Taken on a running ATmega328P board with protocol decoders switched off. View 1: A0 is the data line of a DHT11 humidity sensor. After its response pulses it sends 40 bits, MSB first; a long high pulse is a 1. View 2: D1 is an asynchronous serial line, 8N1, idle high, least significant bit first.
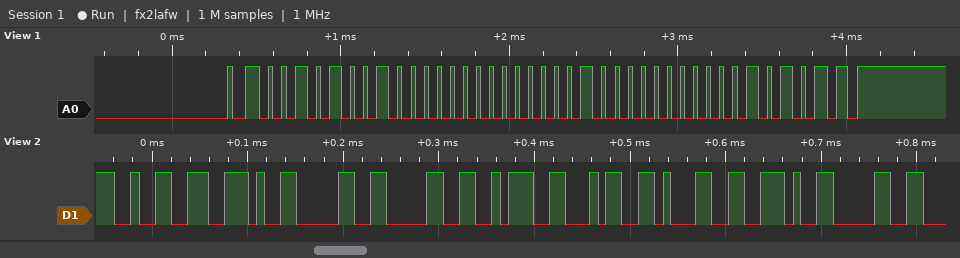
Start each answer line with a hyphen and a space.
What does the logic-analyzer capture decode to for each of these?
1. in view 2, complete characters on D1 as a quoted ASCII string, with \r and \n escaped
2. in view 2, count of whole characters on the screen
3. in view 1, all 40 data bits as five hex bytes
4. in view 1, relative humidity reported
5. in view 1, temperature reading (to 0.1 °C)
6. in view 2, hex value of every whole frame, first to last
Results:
- "2.00:41.0"
- 9
- 29 00 02 00 2B
- 41 %
- 2.0 °C
- 0x32 0x2E 0x30 0x30 0x3A 0x34 0x31 0x2E 0x30
